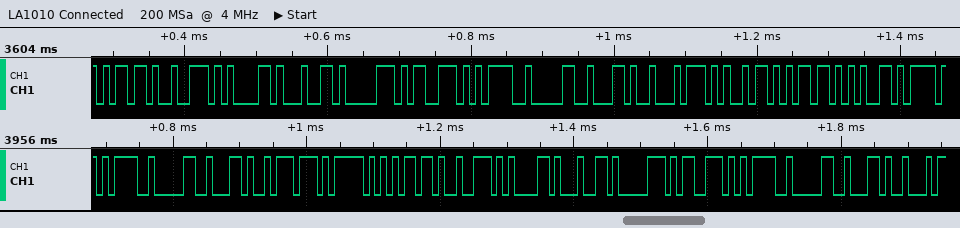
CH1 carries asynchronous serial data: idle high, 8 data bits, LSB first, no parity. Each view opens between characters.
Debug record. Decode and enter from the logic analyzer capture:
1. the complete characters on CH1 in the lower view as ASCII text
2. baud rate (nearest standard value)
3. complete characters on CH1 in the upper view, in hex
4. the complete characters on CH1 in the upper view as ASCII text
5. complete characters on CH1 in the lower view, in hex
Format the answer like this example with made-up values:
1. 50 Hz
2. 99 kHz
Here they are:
1. "=0,w_mradps=0,"
2. 115200 baud
3. 6D, 72, 61, 64, 70, 73, 3D, 30, 2C, 74, 69, 6D, 65
4. "mradps=0,time"
5. 3D, 30, 2C, 77, 5F, 6D, 72, 61, 64, 70, 73, 3D, 30, 2C
